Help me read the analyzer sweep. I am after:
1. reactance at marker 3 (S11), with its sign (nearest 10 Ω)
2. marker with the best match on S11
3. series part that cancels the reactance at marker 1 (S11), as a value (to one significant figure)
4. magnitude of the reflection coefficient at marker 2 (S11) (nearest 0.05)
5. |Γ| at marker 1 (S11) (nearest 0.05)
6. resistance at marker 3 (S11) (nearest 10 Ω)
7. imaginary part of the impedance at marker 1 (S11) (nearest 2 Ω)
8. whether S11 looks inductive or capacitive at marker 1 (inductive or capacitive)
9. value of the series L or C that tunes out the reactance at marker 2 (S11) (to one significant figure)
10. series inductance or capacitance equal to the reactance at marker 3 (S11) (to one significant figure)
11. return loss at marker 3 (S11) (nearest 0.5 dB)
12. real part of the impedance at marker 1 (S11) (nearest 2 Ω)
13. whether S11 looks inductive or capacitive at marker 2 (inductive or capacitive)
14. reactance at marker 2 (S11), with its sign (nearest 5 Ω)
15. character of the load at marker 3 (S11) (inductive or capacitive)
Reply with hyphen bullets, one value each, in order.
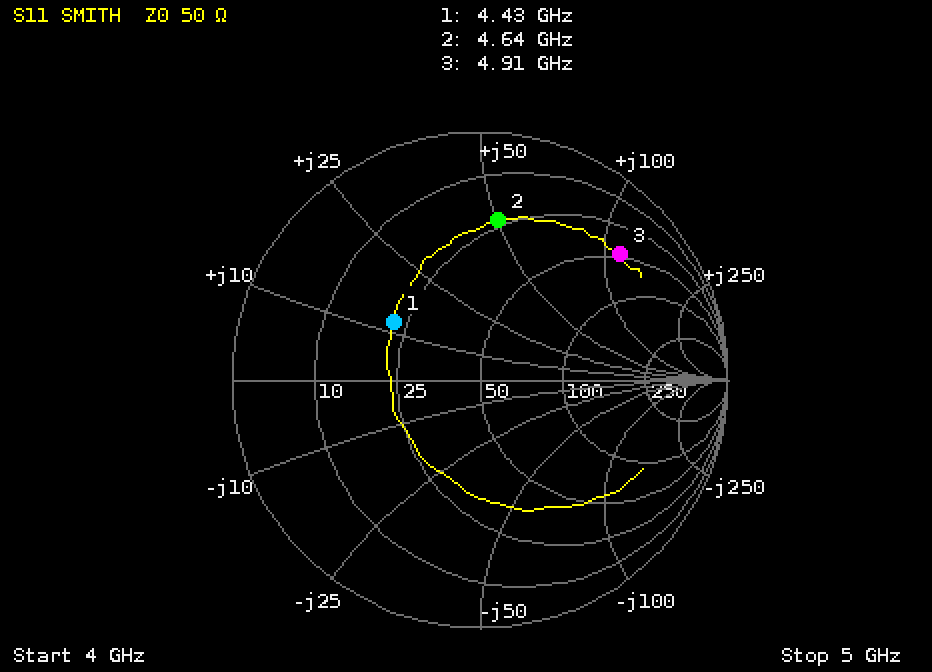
- +110 Ω
- marker 1
- 3 pF
- 0.65
- 0.40
- 50 Ω
- +12 Ω
- inductive
- 700 fF
- 4 nH
- 2.5 dB
- 22 Ω
- inductive
- +50 Ω
- inductive
